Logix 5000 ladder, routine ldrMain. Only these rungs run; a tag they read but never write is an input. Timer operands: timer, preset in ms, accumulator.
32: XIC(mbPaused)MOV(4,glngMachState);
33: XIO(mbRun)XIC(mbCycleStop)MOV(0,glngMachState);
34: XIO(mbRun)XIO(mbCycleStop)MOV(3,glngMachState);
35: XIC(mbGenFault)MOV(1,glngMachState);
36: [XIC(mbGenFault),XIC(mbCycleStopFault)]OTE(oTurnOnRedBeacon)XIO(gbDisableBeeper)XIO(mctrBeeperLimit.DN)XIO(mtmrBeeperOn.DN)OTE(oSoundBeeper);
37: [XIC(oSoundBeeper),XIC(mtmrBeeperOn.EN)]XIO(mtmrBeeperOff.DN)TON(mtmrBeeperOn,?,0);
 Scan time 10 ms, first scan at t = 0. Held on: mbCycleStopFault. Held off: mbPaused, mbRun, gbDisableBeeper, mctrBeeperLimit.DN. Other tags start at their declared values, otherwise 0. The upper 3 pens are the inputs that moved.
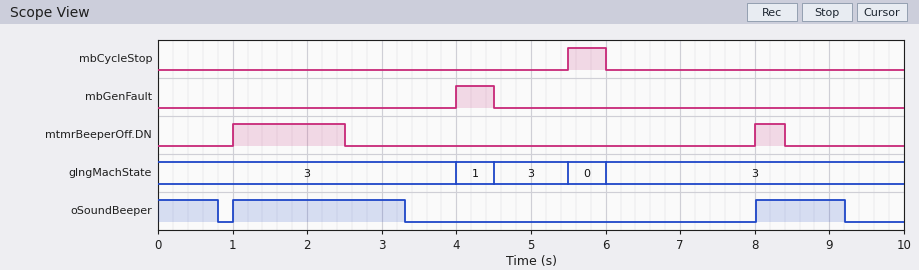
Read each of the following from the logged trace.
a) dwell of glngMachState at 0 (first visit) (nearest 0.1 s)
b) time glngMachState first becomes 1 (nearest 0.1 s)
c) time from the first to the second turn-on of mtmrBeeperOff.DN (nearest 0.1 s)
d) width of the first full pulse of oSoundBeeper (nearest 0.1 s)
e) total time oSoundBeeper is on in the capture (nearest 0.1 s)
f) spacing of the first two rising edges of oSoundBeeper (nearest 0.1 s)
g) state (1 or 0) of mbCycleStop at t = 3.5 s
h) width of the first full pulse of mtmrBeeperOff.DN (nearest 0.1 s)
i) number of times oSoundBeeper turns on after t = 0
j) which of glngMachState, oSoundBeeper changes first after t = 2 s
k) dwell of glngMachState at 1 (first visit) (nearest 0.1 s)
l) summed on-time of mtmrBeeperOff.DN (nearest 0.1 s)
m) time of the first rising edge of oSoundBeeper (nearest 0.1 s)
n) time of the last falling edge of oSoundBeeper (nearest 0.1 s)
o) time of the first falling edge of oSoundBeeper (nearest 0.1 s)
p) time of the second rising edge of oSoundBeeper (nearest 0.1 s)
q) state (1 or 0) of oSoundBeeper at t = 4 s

0.5 s
4.0 s
7.0 s
2.3 s
4.3 s
7.0 s
0
1.5 s
2
oSoundBeeper
0.5 s
1.9 s
1.0 s
9.2 s
0.8 s
8.0 s
0
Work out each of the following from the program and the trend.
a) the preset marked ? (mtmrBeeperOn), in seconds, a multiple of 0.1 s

0.8 s
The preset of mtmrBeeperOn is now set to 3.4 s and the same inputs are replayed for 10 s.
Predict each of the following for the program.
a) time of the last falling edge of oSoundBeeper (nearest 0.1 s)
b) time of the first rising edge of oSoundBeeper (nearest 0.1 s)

5.9 s
8.0 s
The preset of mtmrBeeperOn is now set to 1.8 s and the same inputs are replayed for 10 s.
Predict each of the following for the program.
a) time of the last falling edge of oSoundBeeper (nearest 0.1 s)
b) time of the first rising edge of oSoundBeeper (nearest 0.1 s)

4.3 s
8.0 s
